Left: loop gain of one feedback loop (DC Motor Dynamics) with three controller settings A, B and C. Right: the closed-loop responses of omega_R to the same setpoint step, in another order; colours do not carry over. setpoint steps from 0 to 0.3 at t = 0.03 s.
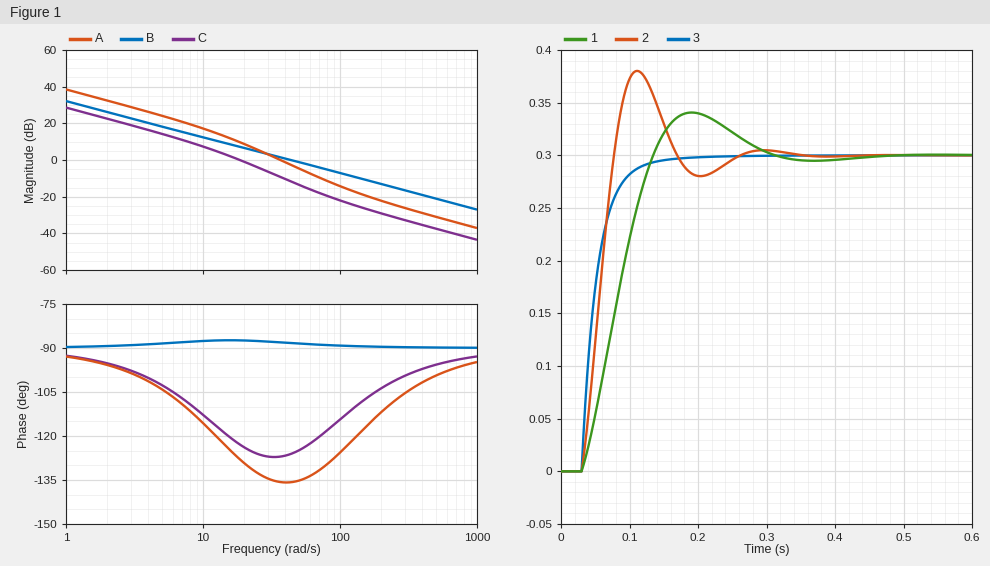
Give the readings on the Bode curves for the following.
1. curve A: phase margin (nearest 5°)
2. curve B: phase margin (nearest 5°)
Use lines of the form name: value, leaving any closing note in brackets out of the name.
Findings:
curve A: phase margin: 45°
curve B: phase margin: 90°
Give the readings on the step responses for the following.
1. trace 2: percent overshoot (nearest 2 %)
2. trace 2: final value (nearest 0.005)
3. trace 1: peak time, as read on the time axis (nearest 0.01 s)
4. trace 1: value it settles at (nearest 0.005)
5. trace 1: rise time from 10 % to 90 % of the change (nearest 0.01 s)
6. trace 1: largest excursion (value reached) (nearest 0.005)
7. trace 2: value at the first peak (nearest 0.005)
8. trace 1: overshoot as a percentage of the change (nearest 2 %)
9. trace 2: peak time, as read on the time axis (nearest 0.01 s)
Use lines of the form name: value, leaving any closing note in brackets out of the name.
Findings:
trace 2: percent overshoot: 26 %
trace 2: final value: 0.300
trace 1: peak time, as read on the time axis: 0.19 s
trace 1: value it settles at: 0.300
trace 1: rise time from 10 % to 90 % of the change: 0.08 s
trace 1: largest excursion (value reached): 0.340
trace 2: value at the first peak: 0.380
trace 1: overshoot as a percentage of the change: 14 %
trace 2: peak time, as read on the time axis: 0.11 s
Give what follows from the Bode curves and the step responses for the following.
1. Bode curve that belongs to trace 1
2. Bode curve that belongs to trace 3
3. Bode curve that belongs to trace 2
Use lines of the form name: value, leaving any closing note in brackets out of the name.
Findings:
Bode curve that belongs to trace 1: C
Bode curve that belongs to trace 3: B
Bode curve that belongs to trace 2: A
